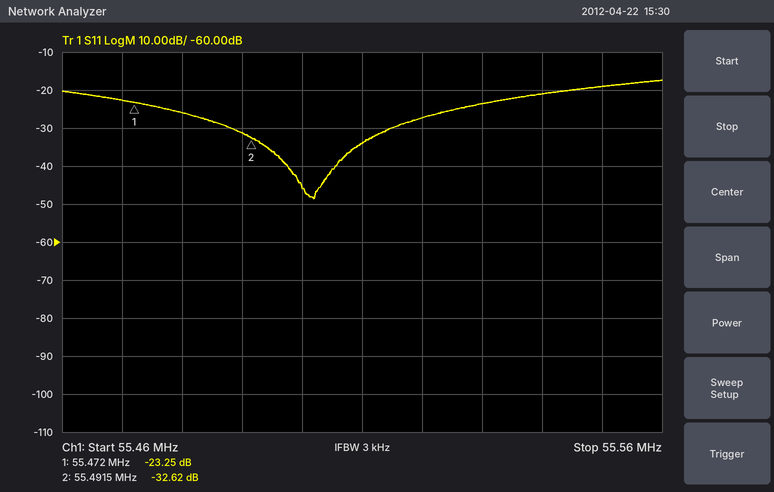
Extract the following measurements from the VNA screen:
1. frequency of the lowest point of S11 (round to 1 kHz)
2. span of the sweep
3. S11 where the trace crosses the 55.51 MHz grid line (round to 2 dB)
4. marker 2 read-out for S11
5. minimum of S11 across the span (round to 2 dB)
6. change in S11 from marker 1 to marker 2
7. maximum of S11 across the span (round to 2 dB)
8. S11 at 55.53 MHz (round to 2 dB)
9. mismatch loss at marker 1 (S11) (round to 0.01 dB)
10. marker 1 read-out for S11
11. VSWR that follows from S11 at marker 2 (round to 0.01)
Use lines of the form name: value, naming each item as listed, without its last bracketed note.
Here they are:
frequency of the lowest point of S11: 55.502 MHz
span of the sweep: 100 kHz
S11 where the trace crosses the 55.51 MHz grid line: -34 dB
marker 2 read-out for S11: -32.62 dB
minimum of S11 across the span: -48 dB
change in S11 from marker 1 to marker 2: -9.37 dB
maximum of S11 across the span: -18 dB
S11 at 55.53 MHz: -24 dB
mismatch loss at marker 1 (S11): 0.02 dB
marker 1 read-out for S11: -23.25 dB
VSWR that follows from S11 at marker 2: 1.05
